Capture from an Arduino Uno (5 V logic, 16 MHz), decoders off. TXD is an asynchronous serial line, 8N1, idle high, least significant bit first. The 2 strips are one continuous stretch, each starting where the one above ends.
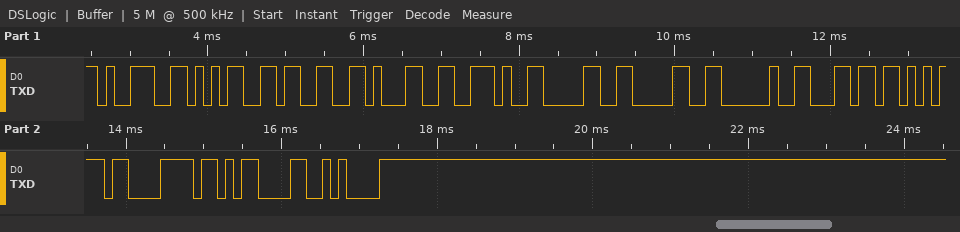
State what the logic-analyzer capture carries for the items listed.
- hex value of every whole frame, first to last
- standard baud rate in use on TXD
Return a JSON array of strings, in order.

["0x39 0x35 0x33 0x31 0x2E 0x30 0x30 0x20 0x6C 0x75 0x78 0x0D 0x0A", "9600 baud"]
